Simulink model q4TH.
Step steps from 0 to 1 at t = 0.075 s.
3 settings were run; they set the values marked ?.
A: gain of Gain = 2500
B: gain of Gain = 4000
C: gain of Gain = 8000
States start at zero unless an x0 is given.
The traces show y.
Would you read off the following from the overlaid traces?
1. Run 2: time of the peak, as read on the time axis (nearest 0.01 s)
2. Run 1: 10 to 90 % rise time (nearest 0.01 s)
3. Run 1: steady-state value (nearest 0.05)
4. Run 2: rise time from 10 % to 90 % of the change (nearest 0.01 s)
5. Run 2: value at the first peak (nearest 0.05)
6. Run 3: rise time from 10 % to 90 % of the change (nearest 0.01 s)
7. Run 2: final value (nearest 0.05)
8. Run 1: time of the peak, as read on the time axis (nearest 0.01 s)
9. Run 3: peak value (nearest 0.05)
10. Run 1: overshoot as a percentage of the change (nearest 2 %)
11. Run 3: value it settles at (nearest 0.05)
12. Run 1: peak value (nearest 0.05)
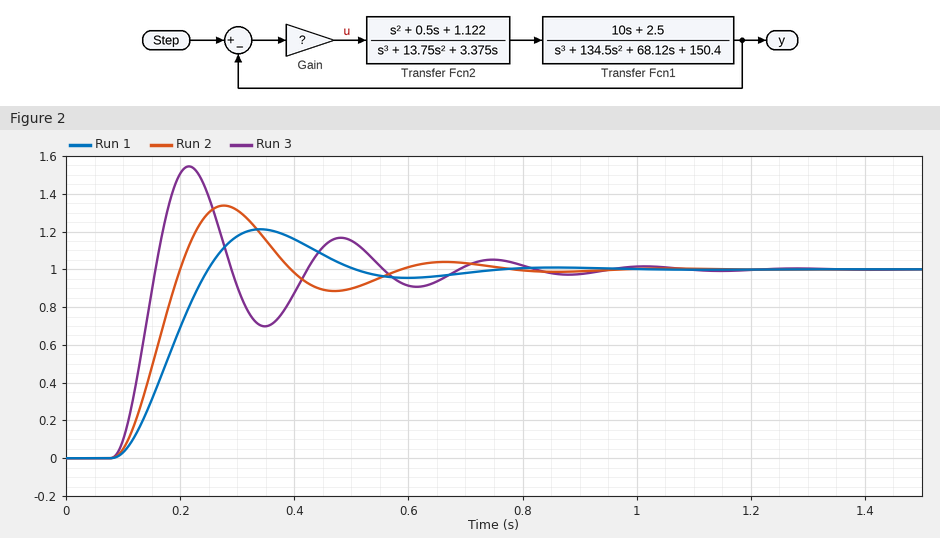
0.28 s
0.11 s
1.00
0.08 s
1.35
0.05 s
1.00
0.34 s
1.55
22 %
1.00
1.20
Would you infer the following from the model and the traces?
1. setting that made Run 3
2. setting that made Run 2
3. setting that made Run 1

C
B
A
